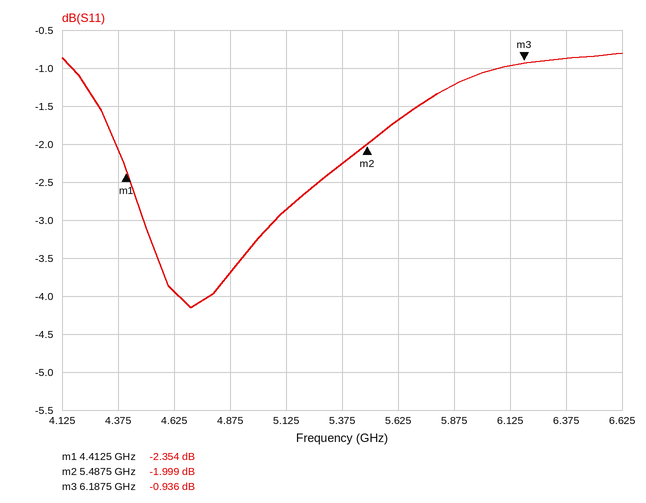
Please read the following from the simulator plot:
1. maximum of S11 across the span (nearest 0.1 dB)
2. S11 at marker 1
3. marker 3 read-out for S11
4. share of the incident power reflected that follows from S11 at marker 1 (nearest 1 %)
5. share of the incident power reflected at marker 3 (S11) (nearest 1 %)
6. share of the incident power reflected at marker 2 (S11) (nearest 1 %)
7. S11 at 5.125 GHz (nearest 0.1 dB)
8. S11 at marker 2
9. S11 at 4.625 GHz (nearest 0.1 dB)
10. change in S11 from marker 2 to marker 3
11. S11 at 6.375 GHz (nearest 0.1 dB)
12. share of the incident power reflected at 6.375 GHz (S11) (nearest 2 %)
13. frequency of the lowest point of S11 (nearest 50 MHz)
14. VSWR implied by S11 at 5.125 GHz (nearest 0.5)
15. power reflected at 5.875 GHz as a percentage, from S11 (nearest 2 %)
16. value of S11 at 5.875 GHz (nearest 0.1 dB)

-0.8 dB
-2.354 dB
-0.936 dB
58 %
81 %
63 %
-2.9 dB
-1.999 dB
-3.9 dB
1.063 dB
-0.9 dB
82 %
4.70 GHz
6.0
76 %
-1.2 dB
